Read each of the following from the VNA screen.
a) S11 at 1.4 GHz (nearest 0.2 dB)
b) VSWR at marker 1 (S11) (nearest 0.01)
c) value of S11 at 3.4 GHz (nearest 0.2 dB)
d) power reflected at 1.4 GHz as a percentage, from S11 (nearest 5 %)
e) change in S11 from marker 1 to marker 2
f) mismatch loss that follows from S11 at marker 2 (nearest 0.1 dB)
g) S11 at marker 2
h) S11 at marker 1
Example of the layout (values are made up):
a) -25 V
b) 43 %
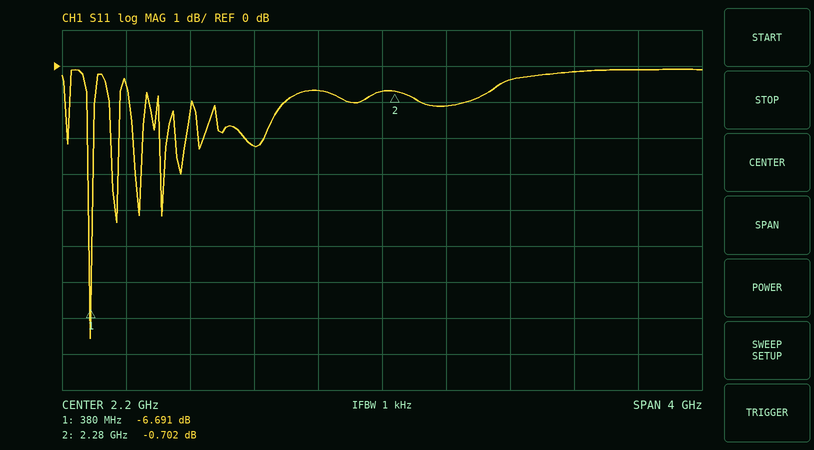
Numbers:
a) -2.2 dB
b) 2.72
c) -0.2 dB
d) 60 %
e) 5.989 dB
f) 8.3 dB
g) -0.702 dB
h) -6.691 dB
